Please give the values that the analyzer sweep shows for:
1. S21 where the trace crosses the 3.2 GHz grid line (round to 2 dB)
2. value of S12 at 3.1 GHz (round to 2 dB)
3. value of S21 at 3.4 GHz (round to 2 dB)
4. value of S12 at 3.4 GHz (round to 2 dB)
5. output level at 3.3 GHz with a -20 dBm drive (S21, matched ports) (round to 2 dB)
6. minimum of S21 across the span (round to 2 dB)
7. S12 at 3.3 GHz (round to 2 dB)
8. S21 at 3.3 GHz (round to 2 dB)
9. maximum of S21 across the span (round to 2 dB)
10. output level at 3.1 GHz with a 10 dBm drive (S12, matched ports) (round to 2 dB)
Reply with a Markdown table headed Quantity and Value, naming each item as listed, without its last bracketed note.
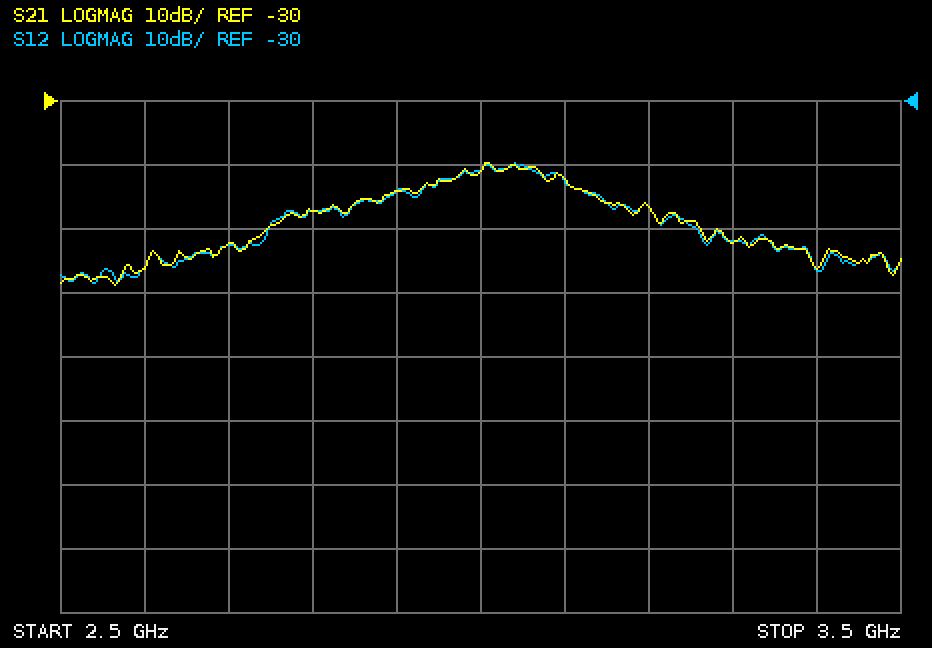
| Quantity | Value |
|---|---|
| S21 where the trace crosses the 3.2 GHz grid line | -46 dB |
| value of S12 at 3.1 GHz | -42 dB |
| value of S21 at 3.4 GHz | -56 dB |
| value of S12 at 3.4 GHz | -56 dB |
| output level at 3.3 GHz with a -20 dBm drive (S21, matched ports) | -72 dBm |
| minimum of S21 across the span | -58 dB |
| S12 at 3.3 GHz | -52 dB |
| S21 at 3.3 GHz | -52 dB |
| maximum of S21 across the span | -40 dB |
| output level at 3.1 GHz with a 10 dBm drive (S12, matched ports) | -32 dBm |
